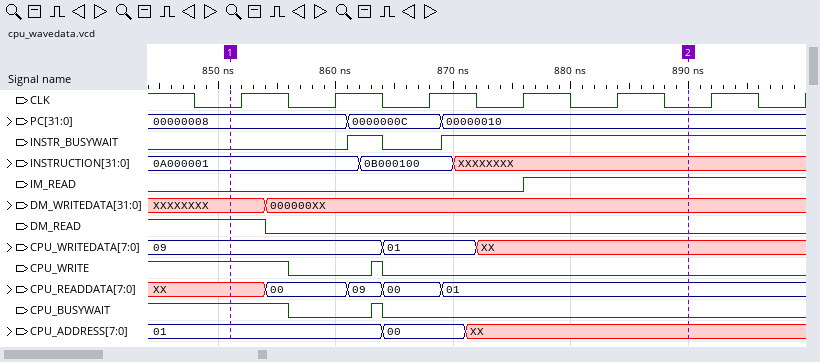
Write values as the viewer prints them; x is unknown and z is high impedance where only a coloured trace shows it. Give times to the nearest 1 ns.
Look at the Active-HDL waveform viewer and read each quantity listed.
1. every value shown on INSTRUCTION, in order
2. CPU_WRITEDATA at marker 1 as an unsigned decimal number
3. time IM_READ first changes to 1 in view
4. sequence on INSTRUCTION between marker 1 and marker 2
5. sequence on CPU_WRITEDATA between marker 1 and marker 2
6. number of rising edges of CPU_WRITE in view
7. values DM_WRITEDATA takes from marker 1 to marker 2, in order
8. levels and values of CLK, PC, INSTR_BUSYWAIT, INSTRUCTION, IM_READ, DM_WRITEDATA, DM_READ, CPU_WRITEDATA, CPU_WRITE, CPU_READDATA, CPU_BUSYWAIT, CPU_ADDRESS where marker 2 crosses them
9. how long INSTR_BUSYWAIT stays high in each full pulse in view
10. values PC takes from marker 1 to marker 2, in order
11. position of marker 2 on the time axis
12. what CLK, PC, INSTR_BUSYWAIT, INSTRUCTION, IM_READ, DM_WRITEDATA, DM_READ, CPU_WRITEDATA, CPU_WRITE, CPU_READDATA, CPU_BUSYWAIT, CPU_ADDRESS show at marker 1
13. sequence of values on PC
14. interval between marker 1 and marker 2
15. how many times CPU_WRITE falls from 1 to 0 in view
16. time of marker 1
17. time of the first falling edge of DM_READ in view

0A000001, 0B000100, XXXXXXXX
9
876 ns
0A000001, 0B000100, XXXXXXXX
09, 01, XX
1
XXXXXXXX, 000000XX
CLK=0, PC=00000010, INSTR_BUSYWAIT=1, INSTRUCTION=XXXXXXXX, IM_READ=1, DM_WRITEDATA=000000XX, DM_READ=0, CPU_WRITEDATA=XX, CPU_WRITE=0, CPU_READDATA=01, CPU_BUSYWAIT=0, CPU_ADDRESS=XX
3 ns
00000008, 0000000C, 00000010
890 ns
CLK=0, PC=00000008, INSTR_BUSYWAIT=0, INSTRUCTION=0A000001, IM_READ=0, DM_WRITEDATA=XXXXXXXX, DM_READ=1, CPU_WRITEDATA=09, CPU_WRITE=1, CPU_READDATA=XX, CPU_BUSYWAIT=1, CPU_ADDRESS=01
00000008, 0000000C, 00000010
39 ns
2
851 ns
854 ns
